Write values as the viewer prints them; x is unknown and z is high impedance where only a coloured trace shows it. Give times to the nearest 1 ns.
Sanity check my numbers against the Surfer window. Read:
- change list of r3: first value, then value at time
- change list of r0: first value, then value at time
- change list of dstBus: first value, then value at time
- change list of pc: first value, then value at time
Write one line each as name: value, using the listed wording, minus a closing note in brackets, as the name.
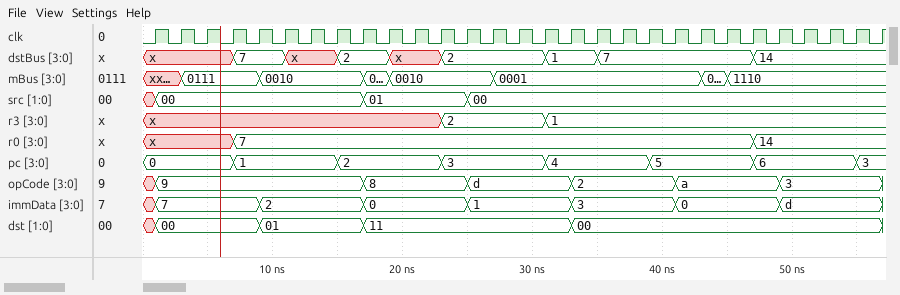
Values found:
change list of r3: first value, then value at time: x, 2 at 23 ns, 1 at 31 ns
change list of r0: first value, then value at time: x, 7 at 7 ns, 14 at 47 ns
change list of dstBus: first value, then value at time: x, 7 at 7 ns, x at 11 ns, 2 at 15 ns, x at 19 ns, 2 at 23 ns, 1 at 31 ns, 7 at 35 ns, 14 at 47 ns
change list of pc: first value, then value at time: 0, 1 at 7 ns, 2 at 15 ns, 3 at 23 ns, 4 at 31 ns, 5 at 39 ns, 6 at 47 ns, 3 at 55 ns
